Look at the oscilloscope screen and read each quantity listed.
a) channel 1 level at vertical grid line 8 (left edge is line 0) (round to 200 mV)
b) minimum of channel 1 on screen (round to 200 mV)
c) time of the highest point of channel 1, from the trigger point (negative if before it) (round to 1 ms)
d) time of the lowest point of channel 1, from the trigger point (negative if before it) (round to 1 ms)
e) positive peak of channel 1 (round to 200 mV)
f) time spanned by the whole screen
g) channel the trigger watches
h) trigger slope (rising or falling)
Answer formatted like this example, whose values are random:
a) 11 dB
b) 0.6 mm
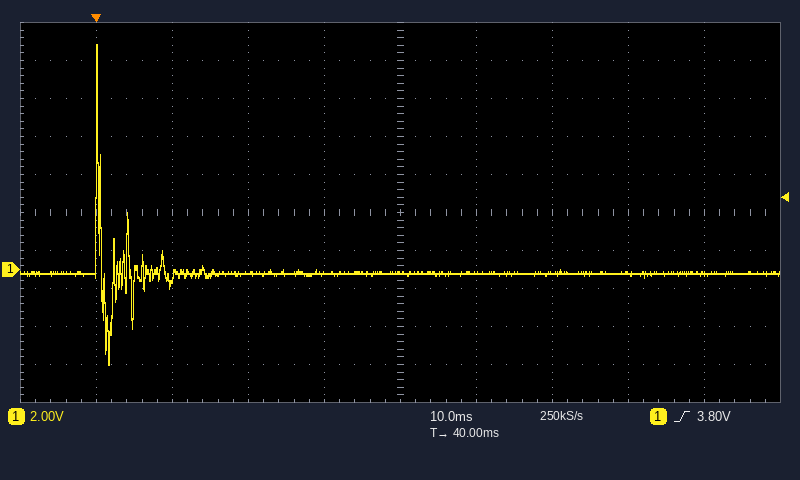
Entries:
a) -200 mV
b) -5.0 V
c) 0 ms
d) +2 ms
e) 11.8 V
f) 100 ms
g) channel 1
h) rising
